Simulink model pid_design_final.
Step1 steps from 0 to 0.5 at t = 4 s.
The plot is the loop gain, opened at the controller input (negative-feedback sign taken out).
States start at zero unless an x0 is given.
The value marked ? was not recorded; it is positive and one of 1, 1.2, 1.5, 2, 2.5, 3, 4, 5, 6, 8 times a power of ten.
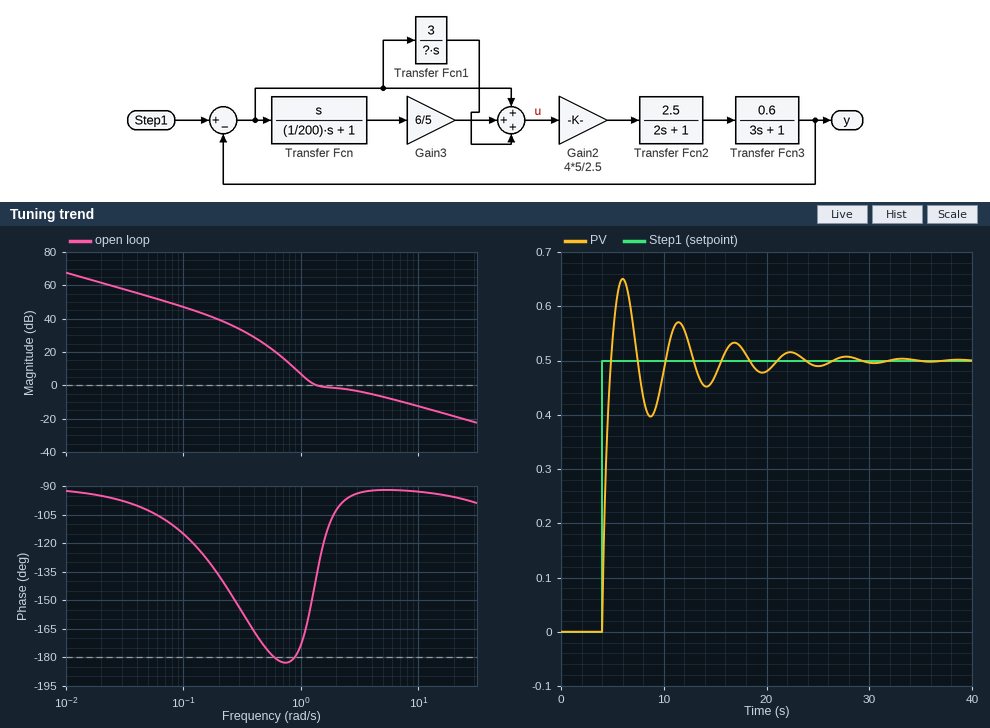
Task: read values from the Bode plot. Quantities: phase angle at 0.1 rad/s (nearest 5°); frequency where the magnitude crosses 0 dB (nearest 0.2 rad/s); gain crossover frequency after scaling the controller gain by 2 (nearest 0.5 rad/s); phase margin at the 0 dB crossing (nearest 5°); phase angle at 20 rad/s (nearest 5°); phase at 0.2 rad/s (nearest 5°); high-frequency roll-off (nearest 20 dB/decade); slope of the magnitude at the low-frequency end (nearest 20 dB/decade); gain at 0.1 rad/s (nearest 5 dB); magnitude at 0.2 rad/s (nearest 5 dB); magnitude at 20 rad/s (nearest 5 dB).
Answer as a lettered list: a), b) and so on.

a) -115°
b) 1.4 rad/s
c) 4.5 rad/s
d) 45°
e) -95°
f) -135°
g) -20 dB/decade
h) -20 dB/decade
i) 45 dB
j) 40 dB
k) -20 dB
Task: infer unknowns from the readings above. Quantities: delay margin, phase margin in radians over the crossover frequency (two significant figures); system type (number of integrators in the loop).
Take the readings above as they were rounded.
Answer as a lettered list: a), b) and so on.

a) 0.56 s
b) 1
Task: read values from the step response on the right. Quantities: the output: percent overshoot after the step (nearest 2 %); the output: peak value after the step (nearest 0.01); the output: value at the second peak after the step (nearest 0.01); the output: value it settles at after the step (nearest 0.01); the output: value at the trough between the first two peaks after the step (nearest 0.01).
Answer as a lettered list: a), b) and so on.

a) 30 %
b) 0.65
c) 0.57
d) 0.50
e) 0.40
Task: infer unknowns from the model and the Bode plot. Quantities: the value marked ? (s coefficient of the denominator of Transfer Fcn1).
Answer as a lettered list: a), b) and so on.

a) 1.5
